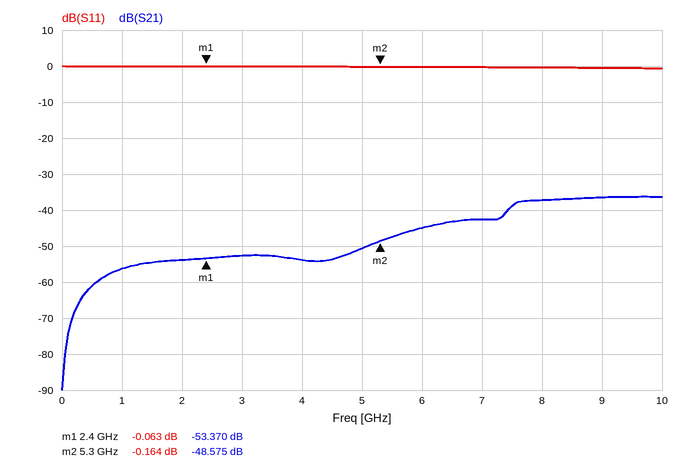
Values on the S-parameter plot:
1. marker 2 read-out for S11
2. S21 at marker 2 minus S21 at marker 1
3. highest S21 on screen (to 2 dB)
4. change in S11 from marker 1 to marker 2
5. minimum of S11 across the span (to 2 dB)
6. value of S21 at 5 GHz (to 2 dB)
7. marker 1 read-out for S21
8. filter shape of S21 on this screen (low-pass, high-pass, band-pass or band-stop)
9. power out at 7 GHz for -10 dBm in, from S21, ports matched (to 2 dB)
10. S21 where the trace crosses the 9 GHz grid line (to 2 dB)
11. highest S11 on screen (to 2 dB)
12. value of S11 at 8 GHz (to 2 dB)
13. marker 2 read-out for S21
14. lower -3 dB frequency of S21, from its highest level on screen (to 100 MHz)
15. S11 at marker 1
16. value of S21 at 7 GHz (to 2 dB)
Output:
-0.164 dB
4.795 dB
-36 dB
-0.101 dB
0 dB
-50 dB
-53.370 dB
high-pass
-52 dBm
-36 dB
0 dB
0 dB
-48.575 dB
7.5 GHz
-0.063 dB
-42 dB
